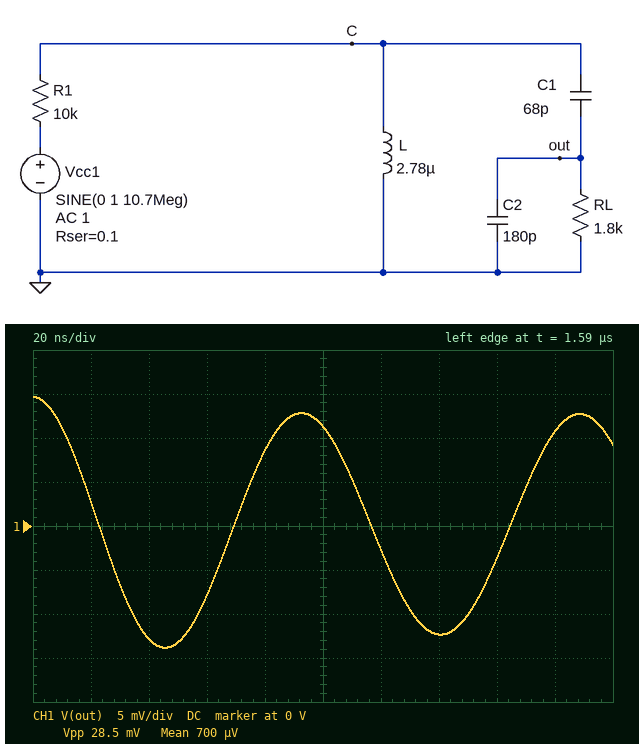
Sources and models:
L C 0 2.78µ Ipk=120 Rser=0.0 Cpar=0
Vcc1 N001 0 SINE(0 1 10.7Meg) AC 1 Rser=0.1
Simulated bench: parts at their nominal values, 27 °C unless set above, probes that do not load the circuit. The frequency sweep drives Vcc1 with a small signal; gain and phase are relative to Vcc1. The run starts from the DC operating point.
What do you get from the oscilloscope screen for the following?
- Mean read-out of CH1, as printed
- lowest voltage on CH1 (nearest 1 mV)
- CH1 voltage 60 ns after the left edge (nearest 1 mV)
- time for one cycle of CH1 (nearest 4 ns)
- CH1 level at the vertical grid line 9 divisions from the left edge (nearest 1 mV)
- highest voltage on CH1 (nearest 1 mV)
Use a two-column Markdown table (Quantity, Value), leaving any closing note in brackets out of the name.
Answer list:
| Quantity | Value |
|---|---|
| Mean read-out of CH1, as printed | 700 µV |
| lowest voltage on CH1 | -14 mV |
| CH1 voltage 60 ns after the left edge | -8 mV |
| time for one cycle of CH1 | 96 ns |
| CH1 level at the vertical grid line 9 divisions from the left edge | 11 mV |
| highest voltage on CH1 | 15 mV |
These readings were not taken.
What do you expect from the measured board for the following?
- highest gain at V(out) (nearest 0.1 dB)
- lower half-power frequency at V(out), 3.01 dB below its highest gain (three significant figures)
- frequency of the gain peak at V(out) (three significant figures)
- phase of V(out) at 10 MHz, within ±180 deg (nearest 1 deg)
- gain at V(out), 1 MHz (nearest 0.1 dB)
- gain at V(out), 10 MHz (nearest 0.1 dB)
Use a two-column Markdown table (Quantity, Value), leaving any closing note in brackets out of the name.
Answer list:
| Quantity | Value |
|---|---|
| highest gain at V(out) | -14.3 dB |
| lower half-power frequency at V(out), 3.01 dB below its highest gain | 13.4 MHz |
| frequency of the gain peak at V(out) | 13.6 MHz |
| phase of V(out) at 10 MHz, within ±180 deg | 89 deg |
| gain at V(out), 1 MHz | -66.9 dB |
| gain at V(out), 10 MHz | -39.6 dB |
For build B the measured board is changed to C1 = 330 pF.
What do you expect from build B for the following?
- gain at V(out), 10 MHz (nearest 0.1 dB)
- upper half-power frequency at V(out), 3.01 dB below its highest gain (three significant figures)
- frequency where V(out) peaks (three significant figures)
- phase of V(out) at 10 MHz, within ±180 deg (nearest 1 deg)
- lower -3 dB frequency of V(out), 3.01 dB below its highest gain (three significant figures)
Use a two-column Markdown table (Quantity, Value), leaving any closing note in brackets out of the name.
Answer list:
| Quantity | Value |
|---|---|
| gain at V(out), 10 MHz | -28.0 dB |
| upper half-power frequency at V(out), 3.01 dB below its highest gain | 9.07 MHz |
| frequency where V(out) peaks | 8.84 MHz |
| phase of V(out) at 10 MHz, within ±180 deg | -77 deg |
| lower -3 dB frequency of V(out), 3.01 dB below its highest gain | 8.62 MHz |
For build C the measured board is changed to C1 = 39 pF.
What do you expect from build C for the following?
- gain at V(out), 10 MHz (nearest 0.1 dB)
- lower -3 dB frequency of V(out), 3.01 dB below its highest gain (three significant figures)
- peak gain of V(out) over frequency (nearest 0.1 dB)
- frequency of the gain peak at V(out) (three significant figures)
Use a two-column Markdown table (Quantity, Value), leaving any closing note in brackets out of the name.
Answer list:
| Quantity | Value |
|---|---|
| gain at V(out), 10 MHz | -46.4 dB |
| lower -3 dB frequency of V(out), 3.01 dB below its highest gain | 16.6 MHz |
| peak gain of V(out) over frequency | -16.4 dB |
| frequency of the gain peak at V(out) | 16.9 MHz |
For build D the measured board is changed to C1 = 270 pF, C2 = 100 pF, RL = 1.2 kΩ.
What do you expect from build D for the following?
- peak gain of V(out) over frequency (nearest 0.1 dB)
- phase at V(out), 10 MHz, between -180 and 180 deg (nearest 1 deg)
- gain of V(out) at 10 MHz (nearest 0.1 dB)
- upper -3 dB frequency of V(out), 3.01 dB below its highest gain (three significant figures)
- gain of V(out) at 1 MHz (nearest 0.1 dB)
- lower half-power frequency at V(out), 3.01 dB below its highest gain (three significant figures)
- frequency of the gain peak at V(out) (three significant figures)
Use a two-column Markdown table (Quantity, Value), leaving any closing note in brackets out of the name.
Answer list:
| Quantity | Value |
|---|---|
| peak gain of V(out) over frequency | -17.4 dB |
| phase at V(out), 10 MHz, between -180 and 180 deg | 66 deg |
| gain of V(out) at 10 MHz | -24.7 dB |
| upper -3 dB frequency of V(out), 3.01 dB below its highest gain | 11.8 MHz |
| gain of V(out) at 1 MHz | -58.3 dB |
| lower half-power frequency at V(out), 3.01 dB below its highest gain | 10.6 MHz |
| frequency of the gain peak at V(out) | 11.2 MHz |
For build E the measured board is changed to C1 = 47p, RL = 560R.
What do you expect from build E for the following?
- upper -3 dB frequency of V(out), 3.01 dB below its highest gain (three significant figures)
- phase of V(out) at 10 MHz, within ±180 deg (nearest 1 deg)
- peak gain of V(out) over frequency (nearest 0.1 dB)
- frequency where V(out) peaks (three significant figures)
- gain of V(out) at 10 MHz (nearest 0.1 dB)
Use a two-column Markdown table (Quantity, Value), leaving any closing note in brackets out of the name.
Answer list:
| Quantity | Value |
|---|---|
| upper -3 dB frequency of V(out), 3.01 dB below its highest gain | 16.0 MHz |
| phase of V(out) at 10 MHz, within ±180 deg | 94 deg |
| peak gain of V(out) over frequency | -18.6 dB |
| frequency where V(out) peaks | 15.6 MHz |
| gain of V(out) at 10 MHz | -44.3 dB |
